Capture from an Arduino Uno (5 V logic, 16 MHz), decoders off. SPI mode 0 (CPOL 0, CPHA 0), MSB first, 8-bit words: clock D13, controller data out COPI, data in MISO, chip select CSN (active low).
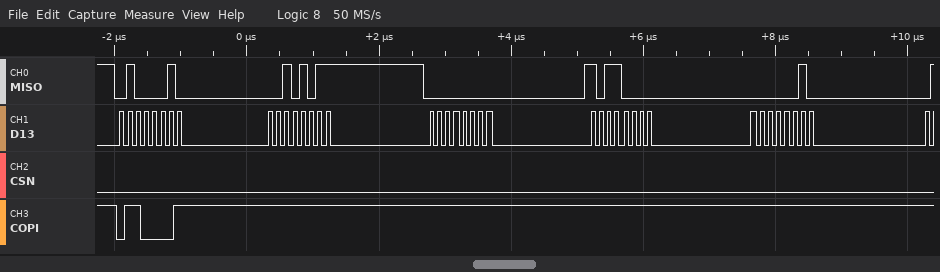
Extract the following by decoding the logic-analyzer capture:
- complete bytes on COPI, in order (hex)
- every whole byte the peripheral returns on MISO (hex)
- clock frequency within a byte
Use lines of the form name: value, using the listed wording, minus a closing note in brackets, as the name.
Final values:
complete bytes on COPI, in order: 61 FF FF FF FF
every whole byte the peripheral returns on MISO: 42 2B 00 B0 02
clock frequency within a byte: 8 MHz
